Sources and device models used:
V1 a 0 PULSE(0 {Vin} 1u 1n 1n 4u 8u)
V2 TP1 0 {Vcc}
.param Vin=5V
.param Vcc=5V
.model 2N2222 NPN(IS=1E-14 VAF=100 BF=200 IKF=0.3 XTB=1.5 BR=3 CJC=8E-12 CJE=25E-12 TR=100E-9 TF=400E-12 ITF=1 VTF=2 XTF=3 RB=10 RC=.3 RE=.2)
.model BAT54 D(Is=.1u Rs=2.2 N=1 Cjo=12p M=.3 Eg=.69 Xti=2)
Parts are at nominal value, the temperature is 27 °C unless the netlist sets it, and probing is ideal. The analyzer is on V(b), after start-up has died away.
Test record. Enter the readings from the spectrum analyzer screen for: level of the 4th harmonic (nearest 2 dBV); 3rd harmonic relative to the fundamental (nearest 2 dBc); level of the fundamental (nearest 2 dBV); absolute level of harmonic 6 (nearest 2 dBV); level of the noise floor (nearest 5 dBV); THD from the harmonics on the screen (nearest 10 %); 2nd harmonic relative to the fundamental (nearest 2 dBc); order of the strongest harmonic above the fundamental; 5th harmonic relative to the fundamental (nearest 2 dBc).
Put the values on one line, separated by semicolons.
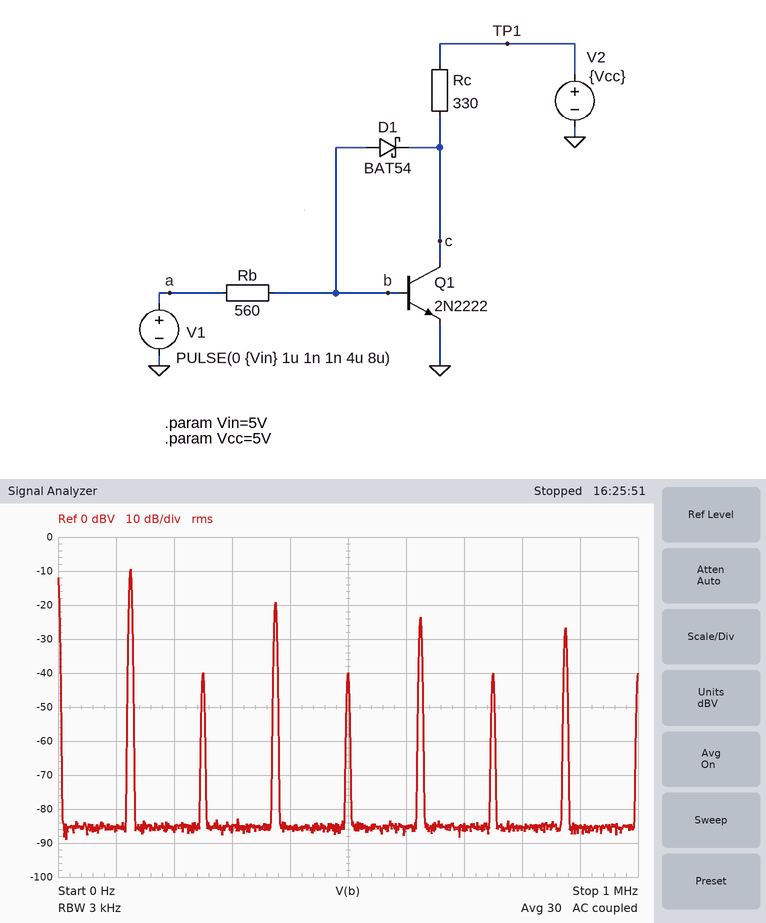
-40 dBV; -10 dBc; -10 dBV; -40 dBV; -85 dBV; 40 %; -30 dBc; 3; -14 dBc
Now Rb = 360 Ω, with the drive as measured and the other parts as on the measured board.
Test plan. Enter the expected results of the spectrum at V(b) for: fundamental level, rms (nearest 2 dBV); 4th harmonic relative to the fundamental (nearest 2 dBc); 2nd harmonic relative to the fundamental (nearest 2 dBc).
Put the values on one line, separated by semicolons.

-10 dBV; -34 dBc; -34 dBc
